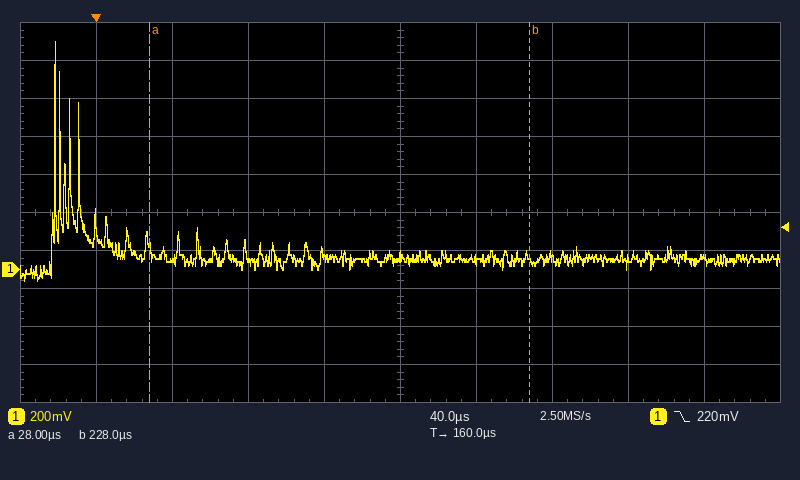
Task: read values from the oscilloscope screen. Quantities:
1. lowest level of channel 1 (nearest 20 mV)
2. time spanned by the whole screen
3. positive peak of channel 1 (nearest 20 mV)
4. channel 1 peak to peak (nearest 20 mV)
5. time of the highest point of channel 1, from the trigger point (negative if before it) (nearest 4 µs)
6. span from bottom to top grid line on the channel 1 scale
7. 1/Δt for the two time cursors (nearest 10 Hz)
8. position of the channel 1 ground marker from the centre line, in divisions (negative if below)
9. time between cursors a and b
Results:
-60 mV
400 µs
1.20 V
1.26 V
-20 µs
2 V
5.00 kHz
-1.5 div
200 µs
